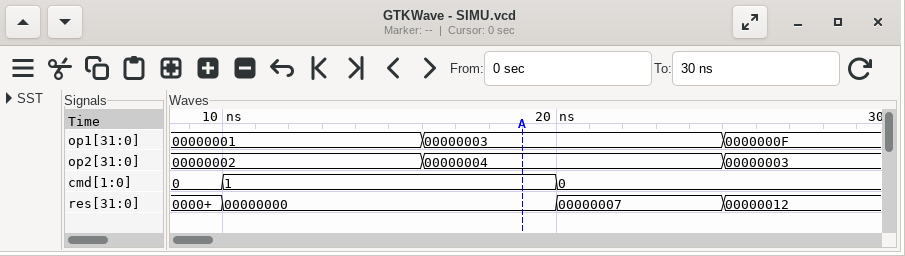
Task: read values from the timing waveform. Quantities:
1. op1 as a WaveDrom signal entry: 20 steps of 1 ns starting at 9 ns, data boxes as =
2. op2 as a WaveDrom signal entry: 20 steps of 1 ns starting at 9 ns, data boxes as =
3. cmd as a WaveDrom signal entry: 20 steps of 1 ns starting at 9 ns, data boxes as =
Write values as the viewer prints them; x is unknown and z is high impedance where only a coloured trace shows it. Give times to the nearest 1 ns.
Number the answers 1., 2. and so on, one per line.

1. {name: 'op1', wave: '=......=........=...', data: '00000001 00000003 0000000F'}
2. {name: 'op2', wave: '=......=........=...', data: '00000002 00000004 00000003'}
3. {name: 'cmd', wave: '==.........=........', data: '0 1 0'}
